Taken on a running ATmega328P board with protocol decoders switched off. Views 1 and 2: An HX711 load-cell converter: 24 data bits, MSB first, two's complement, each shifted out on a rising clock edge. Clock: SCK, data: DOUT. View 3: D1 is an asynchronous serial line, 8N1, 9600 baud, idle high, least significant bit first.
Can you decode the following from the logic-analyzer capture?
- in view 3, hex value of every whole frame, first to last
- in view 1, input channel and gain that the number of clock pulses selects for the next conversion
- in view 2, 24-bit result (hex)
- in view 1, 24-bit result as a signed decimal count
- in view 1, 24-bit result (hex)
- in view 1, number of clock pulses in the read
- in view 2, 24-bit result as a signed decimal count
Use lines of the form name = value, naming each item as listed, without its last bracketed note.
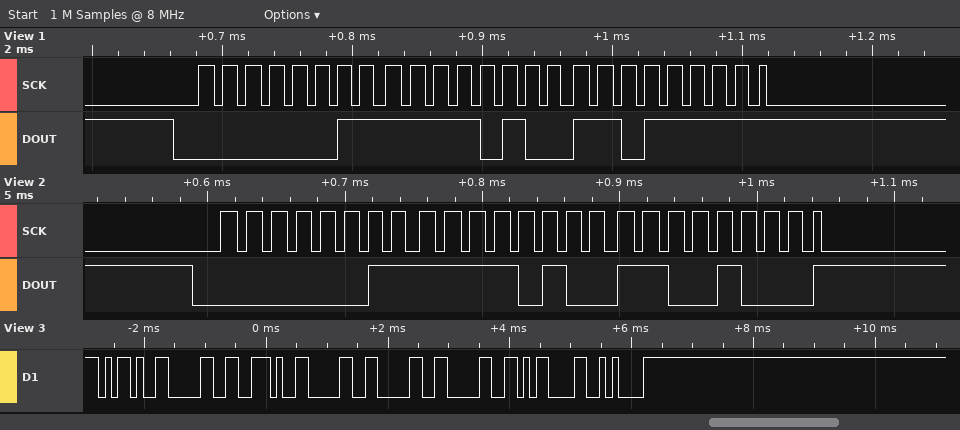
in view 3, hex value of every whole frame, first to last = 2D 30 2E 30 30 30 0D 0A
in view 1, input channel and gain that the number of clock pulses selects for the next conversion = channel A, gain 128
in view 2, 24-bit result = 0x03F4C8
in view 1, 24-bit result as a signed decimal count = 259295
in view 1, 24-bit result = 0x03F4DF
in view 1, number of clock pulses in the read = 25
in view 2, 24-bit result as a signed decimal count = 259272
